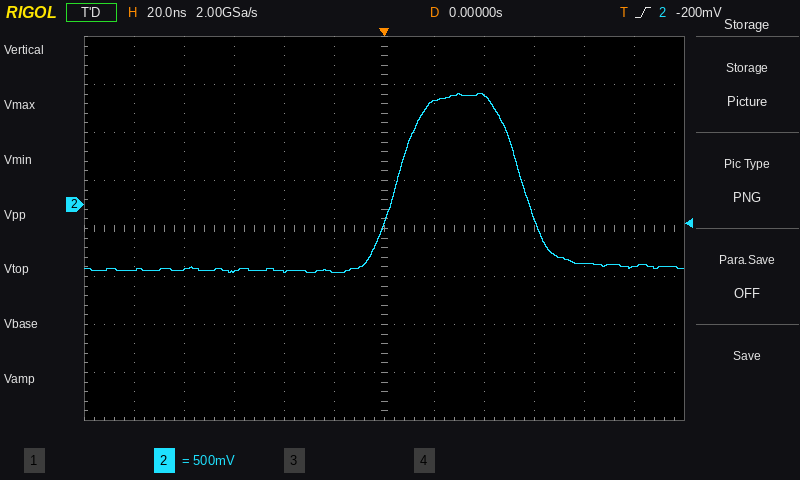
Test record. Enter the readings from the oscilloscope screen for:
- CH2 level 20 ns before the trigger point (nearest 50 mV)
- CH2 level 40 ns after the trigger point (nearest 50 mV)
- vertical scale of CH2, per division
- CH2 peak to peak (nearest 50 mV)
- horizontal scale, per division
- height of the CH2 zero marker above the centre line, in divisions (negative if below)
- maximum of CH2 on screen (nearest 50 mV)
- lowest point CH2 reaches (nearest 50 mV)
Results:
-700 mV
1.15 V
500 mV
1.85 V
20 ns
+0.5 div
1.15 V
-700 mV
